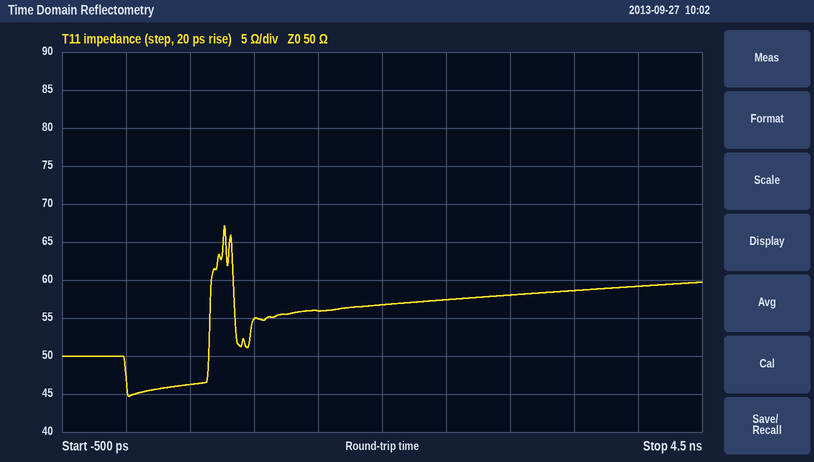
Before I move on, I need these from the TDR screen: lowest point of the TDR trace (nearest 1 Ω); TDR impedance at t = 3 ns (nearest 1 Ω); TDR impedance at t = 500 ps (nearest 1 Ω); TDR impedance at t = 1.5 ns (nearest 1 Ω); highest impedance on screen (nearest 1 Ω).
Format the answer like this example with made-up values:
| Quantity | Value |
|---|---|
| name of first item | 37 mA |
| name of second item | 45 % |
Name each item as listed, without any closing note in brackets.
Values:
| Quantity | Value |
|---|---|
| lowest point of the TDR trace | 45 Ω |
| TDR impedance at t = 3 ns | 58 Ω |
| TDR impedance at t = 500 ps | 46 Ω |
| TDR impedance at t = 1.5 ns | 56 Ω |
| highest impedance on screen | 67 Ω |
